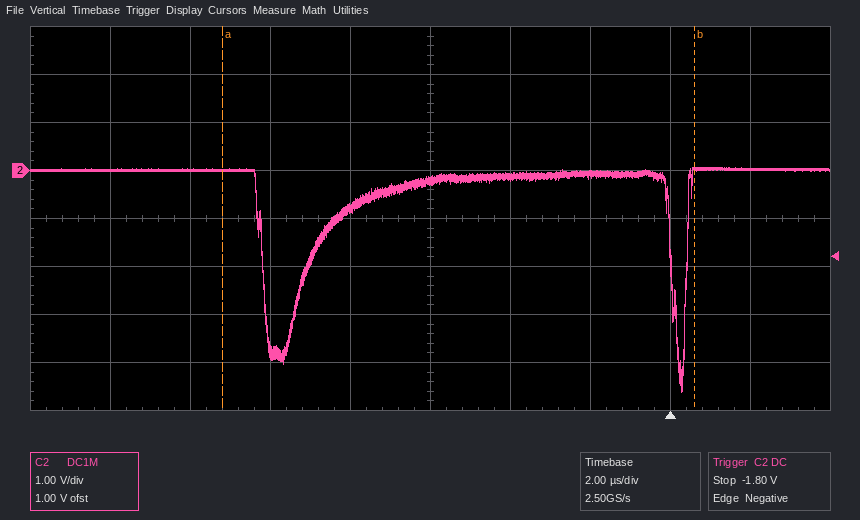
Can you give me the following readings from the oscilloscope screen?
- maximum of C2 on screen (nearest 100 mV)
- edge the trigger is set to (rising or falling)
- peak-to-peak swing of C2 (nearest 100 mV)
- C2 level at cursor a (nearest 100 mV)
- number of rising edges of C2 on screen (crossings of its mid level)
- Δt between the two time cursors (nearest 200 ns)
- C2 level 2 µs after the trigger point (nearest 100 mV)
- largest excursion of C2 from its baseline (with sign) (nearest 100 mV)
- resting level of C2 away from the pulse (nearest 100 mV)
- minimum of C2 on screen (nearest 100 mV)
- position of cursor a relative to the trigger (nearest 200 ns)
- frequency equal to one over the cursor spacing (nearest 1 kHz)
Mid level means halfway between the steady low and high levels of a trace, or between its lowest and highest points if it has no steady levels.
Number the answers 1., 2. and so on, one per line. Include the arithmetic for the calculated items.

1. 100 mV
2. falling
3. 100 mV − (-4.6 V) = 4.7 V
4. 0.0 V
5. 2
6. 11.8 µs
7. 0.0 V
8. -4.6 V − (0.0 V) = -4.6 V
9. 0.0 V
10. -4.6 V
11. -11.2 µs
12. 1 / 11.8 µs ≈ 85 kHz
